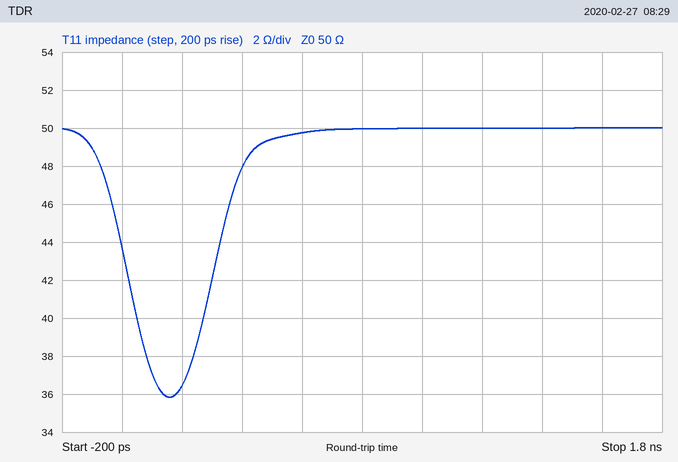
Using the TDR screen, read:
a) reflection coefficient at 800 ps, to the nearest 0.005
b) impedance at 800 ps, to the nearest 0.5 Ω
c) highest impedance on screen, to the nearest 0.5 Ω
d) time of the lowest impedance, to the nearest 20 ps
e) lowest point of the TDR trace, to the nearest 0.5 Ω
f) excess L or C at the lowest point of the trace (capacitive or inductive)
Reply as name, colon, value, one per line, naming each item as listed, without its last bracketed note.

reflection coefficient at 800 ps, to the nearest 0.005: 0.000
impedance at 800 ps, to the nearest 0.5 Ω: 50.0 Ω
highest impedance on screen, to the nearest 0.5 Ω: 50.0 Ω
time of the lowest impedance, to the nearest 20 ps: 160 ps
lowest point of the TDR trace, to the nearest 0.5 Ω: 36.0 Ω
excess L or C at the lowest point of the trace: capacitive
